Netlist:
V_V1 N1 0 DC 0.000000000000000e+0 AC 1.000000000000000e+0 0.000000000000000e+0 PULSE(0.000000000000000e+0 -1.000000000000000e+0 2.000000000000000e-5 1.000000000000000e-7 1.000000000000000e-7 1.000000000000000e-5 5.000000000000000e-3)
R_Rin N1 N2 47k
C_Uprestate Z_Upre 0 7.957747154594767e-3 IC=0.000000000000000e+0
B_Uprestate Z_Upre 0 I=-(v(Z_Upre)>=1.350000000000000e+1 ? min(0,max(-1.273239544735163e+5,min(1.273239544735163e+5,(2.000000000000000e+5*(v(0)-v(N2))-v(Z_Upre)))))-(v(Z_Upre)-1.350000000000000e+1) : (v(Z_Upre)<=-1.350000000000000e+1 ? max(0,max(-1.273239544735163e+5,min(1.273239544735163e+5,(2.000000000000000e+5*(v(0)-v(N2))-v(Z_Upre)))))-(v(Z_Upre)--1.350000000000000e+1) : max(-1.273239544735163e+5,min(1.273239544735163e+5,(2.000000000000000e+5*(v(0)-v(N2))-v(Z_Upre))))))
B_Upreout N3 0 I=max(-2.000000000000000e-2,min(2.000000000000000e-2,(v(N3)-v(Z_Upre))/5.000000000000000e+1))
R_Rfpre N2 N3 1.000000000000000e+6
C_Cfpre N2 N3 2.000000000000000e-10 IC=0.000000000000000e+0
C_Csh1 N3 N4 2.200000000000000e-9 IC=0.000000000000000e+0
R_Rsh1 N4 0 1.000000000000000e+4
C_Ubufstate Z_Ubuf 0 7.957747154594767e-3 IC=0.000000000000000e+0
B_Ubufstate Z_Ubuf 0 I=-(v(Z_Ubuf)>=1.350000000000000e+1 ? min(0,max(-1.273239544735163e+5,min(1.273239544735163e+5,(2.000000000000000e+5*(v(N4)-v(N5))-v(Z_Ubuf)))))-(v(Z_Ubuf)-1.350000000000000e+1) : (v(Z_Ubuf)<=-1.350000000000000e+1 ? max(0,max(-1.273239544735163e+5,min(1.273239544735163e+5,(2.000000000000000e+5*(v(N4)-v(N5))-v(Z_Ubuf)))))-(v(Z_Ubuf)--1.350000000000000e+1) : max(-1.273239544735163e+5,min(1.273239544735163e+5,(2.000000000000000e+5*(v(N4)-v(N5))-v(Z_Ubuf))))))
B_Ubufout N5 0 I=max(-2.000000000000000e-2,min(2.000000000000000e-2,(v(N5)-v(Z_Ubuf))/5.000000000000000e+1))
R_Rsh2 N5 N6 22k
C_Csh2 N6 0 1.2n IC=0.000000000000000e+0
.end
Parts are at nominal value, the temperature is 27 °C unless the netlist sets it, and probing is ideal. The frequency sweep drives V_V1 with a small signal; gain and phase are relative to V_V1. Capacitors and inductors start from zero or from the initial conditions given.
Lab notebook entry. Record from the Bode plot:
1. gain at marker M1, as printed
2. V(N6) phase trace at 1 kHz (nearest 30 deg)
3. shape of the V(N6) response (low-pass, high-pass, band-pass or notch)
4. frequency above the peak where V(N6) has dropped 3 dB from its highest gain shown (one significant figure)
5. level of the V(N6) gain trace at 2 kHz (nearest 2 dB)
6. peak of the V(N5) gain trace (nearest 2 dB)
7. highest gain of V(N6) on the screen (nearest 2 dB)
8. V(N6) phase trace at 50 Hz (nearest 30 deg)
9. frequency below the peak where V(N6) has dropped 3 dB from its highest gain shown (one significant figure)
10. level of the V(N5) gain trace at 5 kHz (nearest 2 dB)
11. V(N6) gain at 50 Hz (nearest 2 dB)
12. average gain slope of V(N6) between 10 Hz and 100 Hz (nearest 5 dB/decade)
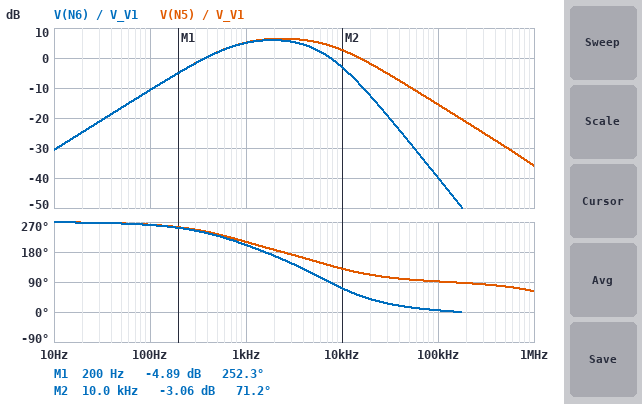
-4.89 dB
210 deg
band-pass
5 kHz
6 dB
6 dB
6 dB
270 deg
600 Hz
6 dB
-16 dB
20 dB/decade
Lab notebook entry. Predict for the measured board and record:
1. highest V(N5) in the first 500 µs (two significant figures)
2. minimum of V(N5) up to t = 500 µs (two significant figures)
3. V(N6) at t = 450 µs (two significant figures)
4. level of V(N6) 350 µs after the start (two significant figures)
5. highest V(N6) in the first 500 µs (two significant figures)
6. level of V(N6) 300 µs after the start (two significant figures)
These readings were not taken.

830 mV
-68 mV
-18 mV
-30 mV
330 mV
-38 mV
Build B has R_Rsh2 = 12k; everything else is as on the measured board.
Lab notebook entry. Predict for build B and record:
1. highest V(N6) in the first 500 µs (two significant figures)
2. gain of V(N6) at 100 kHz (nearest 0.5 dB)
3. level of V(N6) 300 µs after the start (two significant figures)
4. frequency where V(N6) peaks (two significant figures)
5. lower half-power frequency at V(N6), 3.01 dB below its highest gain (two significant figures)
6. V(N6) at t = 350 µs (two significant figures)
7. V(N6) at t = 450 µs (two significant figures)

440 mV
-34.5 dB
-36 mV
2.2 kHz
640 Hz
-28 mV
-17 mV
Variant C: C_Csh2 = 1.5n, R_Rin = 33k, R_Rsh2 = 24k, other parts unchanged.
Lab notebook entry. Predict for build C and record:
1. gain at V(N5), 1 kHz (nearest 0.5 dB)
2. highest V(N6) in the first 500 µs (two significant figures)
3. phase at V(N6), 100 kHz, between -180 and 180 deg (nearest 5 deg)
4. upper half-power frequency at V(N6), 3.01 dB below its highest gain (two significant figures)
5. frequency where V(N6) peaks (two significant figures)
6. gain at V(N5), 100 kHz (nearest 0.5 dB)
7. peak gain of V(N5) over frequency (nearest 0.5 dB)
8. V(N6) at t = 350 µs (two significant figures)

8.0 dB
390 mV
5 deg
4.5 kHz
1.7 kHz
-12.5 dB
9.5 dB
-45 mV
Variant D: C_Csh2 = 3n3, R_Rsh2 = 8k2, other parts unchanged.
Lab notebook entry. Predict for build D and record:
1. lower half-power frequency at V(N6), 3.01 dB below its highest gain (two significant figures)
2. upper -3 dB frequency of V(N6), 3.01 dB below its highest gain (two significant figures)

600 Hz
5.2 kHz
